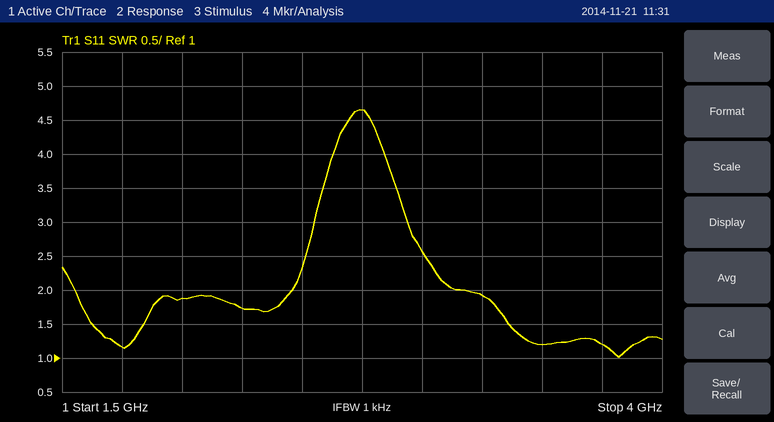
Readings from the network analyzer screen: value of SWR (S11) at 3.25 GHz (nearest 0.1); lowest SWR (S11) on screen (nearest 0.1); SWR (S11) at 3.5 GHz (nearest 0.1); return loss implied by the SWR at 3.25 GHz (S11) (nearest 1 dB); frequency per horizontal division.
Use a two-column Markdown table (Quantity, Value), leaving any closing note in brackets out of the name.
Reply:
| Quantity | Value |
|---|---|
| value of SWR (S11) at 3.25 GHz | 1.9 |
| lowest SWR (S11) on screen | 1.0 |
| SWR (S11) at 3.5 GHz | 1.2 |
| return loss implied by the SWR at 3.25 GHz (S11) | 10 dB |
| frequency per horizontal division | 250 MHz |
